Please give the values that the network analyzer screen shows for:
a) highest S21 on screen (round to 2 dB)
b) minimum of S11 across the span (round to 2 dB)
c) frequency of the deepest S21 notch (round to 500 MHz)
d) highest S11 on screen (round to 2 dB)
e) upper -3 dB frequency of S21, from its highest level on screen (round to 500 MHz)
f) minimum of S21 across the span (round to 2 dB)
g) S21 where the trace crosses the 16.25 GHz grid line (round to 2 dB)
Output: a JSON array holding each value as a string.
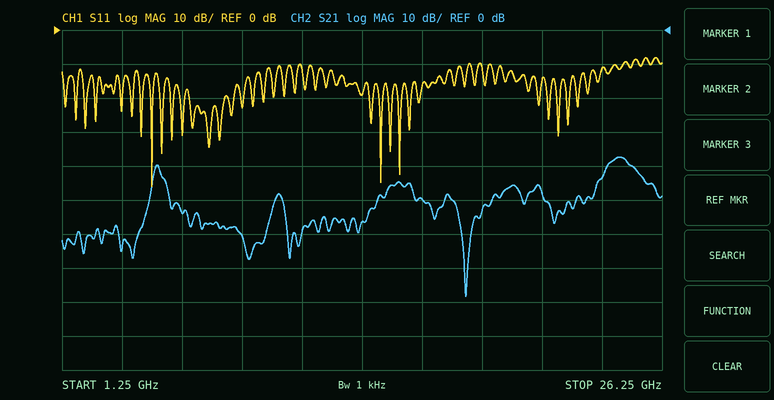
["-38 dB", "-46 dB", "18.0 GHz", "-8 dB", "25.0 GHz", "-78 dB", "-50 dB"]
